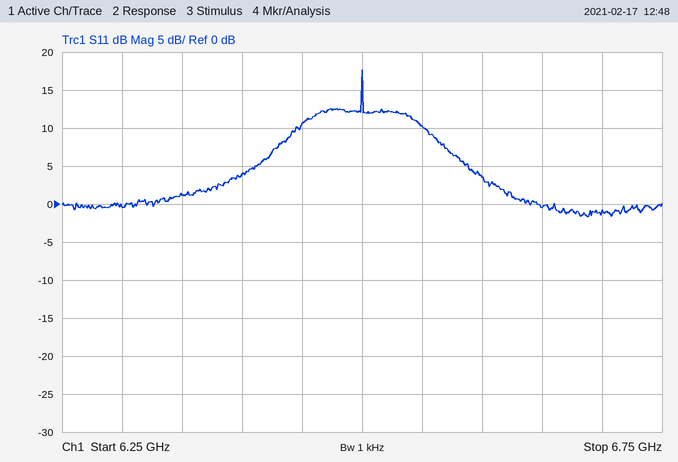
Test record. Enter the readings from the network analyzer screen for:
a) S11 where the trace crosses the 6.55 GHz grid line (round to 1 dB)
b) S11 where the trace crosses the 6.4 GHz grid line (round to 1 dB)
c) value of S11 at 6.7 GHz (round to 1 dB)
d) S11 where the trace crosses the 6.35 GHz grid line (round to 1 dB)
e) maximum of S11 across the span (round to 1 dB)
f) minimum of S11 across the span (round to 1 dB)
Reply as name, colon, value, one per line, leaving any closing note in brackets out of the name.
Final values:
S11 where the trace crosses the 6.55 GHz grid line: 10 dB
S11 where the trace crosses the 6.4 GHz grid line: 4 dB
value of S11 at 6.7 GHz: -1 dB
S11 where the trace crosses the 6.35 GHz grid line: 1 dB
maximum of S11 across the span: 18 dB
minimum of S11 across the span: -2 dB
